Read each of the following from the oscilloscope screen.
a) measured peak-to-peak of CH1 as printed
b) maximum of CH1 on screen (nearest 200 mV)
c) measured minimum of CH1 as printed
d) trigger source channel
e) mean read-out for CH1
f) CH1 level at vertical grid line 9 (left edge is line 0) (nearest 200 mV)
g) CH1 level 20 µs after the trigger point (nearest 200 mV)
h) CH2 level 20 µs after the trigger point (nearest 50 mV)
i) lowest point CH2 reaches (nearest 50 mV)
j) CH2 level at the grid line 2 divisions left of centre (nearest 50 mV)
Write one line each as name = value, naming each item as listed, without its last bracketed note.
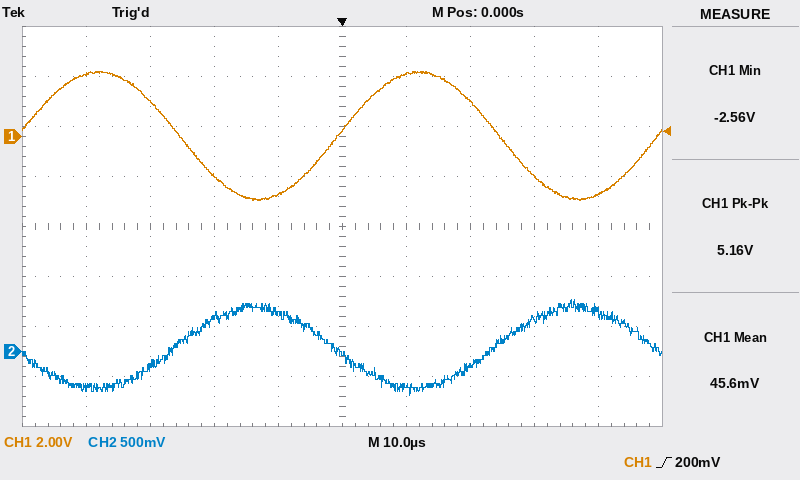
measured peak-to-peak of CH1 as printed = 5.16 V
maximum of CH1 on screen = 2.6 V
measured minimum of CH1 as printed = -2.56 V
trigger source channel = CH1
mean read-out for CH1 = 45.6 mV
CH1 level at vertical grid line 9 (left edge is line 0) = -2.4 V
CH1 level 20 µs after the trigger point = 1.4 V
CH2 level 20 µs after the trigger point = -150 mV
lowest point CH2 reaches = -450 mV
CH2 level at the grid line 2 divisions left of centre = 350 mV
